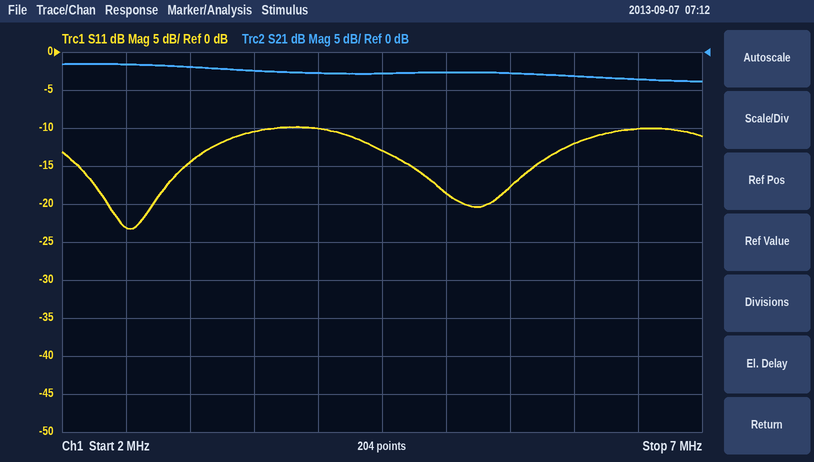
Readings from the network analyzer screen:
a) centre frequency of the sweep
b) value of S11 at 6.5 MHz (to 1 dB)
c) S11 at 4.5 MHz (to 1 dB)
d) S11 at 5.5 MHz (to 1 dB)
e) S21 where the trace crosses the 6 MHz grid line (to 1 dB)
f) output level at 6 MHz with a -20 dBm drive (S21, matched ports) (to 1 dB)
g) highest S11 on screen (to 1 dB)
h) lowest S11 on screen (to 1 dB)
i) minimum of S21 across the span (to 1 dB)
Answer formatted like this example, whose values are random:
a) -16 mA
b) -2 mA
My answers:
a) 4.5 MHz
b) -10 dB
c) -13 dB
d) -18 dB
e) -3 dB
f) -23 dBm
g) -10 dB
h) -23 dB
i) -4 dB
